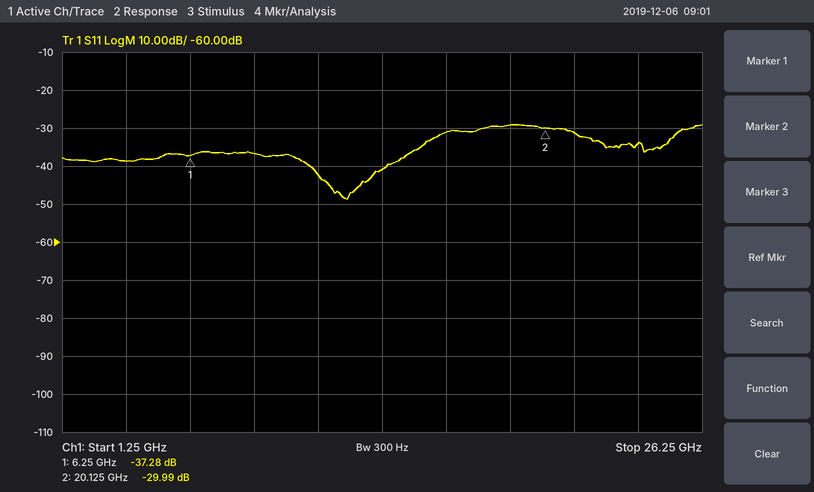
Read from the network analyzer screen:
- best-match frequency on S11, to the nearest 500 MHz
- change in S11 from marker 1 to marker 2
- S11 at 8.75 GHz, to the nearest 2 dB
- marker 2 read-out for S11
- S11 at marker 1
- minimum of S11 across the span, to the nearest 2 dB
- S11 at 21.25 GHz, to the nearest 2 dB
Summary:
12.5 GHz
7.29 dB
-36 dB
-29.99 dB
-37.28 dB
-48 dB
-32 dB
